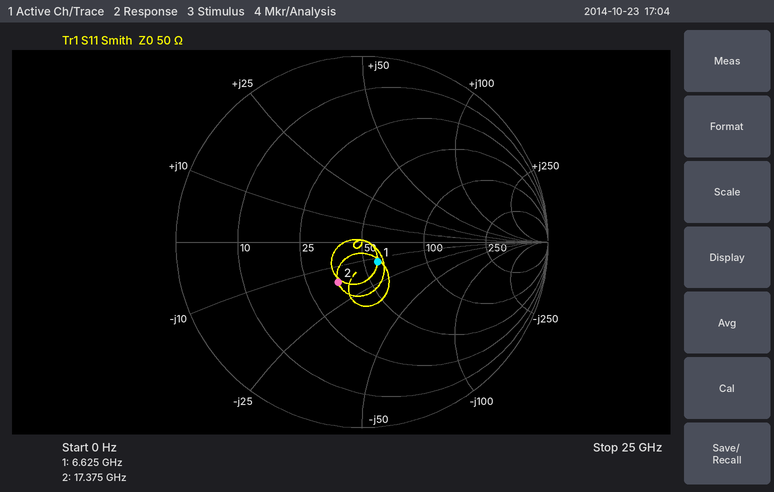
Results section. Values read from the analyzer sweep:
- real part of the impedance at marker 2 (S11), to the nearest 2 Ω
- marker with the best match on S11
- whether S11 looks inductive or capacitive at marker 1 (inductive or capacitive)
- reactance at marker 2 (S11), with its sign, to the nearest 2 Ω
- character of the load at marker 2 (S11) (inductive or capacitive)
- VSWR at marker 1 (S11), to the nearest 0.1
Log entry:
36 Ω
marker 1
capacitive
-16 Ω
capacitive
1.3
